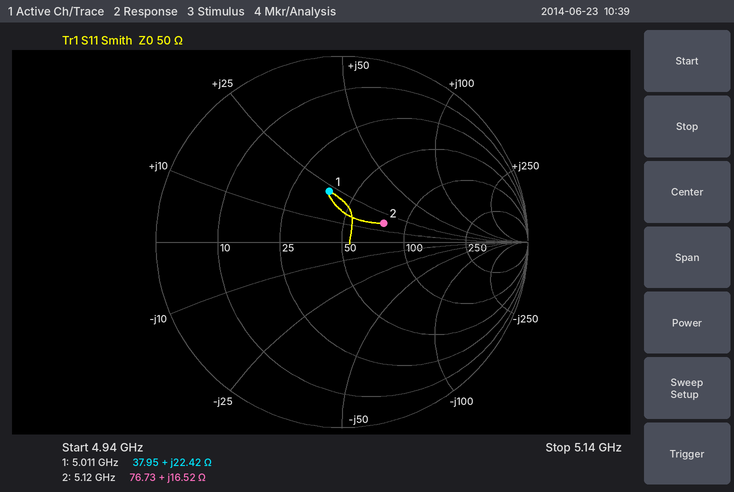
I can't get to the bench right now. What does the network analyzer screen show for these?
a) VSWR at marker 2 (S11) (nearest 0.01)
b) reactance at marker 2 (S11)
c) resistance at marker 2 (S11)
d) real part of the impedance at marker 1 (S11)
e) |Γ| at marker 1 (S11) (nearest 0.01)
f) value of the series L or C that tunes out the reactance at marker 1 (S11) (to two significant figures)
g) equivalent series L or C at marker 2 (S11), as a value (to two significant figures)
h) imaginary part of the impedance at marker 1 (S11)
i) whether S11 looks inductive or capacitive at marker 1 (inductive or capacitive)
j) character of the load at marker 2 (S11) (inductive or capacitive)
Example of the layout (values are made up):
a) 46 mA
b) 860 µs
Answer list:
a) 1.65
b) +16.52 Ω
c) 76.73 Ω
d) 37.95 Ω
e) 0.28
f) 1.4 pF
g) 510 pH
h) +22.42 Ω
i) inductive
j) inductive
